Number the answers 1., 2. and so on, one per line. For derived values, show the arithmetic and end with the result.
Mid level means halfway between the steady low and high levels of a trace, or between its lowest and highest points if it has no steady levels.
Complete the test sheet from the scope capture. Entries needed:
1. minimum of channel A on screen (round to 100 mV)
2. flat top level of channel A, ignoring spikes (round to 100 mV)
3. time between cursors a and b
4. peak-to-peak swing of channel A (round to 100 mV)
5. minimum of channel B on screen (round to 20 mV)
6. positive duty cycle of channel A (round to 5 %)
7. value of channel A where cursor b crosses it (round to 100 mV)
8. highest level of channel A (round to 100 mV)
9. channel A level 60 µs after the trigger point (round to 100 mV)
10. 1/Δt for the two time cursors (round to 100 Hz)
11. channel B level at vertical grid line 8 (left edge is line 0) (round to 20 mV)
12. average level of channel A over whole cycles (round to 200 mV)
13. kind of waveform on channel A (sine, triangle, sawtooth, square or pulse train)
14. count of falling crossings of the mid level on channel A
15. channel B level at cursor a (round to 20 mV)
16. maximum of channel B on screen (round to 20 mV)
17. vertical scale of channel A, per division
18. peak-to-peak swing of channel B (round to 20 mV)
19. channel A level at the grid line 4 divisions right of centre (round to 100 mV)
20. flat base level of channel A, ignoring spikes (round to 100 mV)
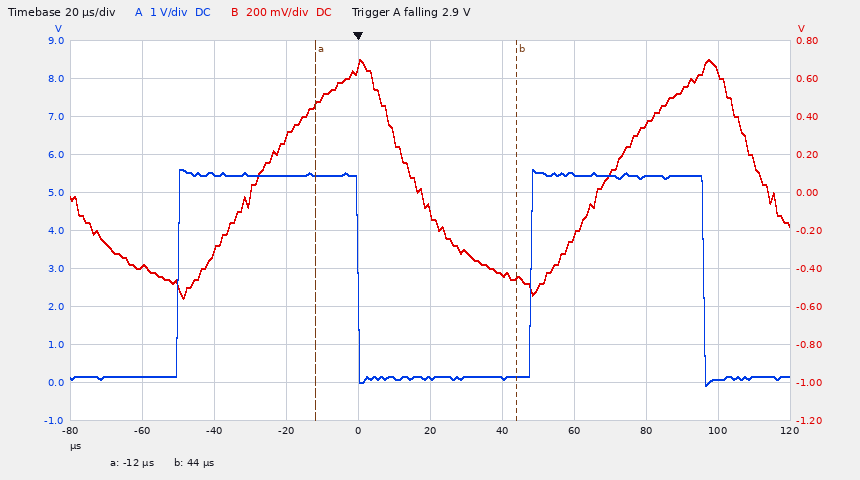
1. -100 mV
2. 5.4 V
3. 44 µs − (-12 µs) = 56 µs
4. 5.6 V − (-100 mV) = 5.7 V
5. -560 mV
6. 50 %
7. 200 mV
8. 5.6 V
9. 5.5 V
10. 1 / 56 µs ≈ 17.9 kHz
11. 360 mV
12. 200 mV + 0.5 × (5.4 V − (200 mV)) ≈ 2.8 V
13. square
14. 2
15. 460 mV
16. 700 mV
17. 1 V
18. 700 mV − (-560 mV) = 1.26 V
19. 100 mV
20. 200 mV
